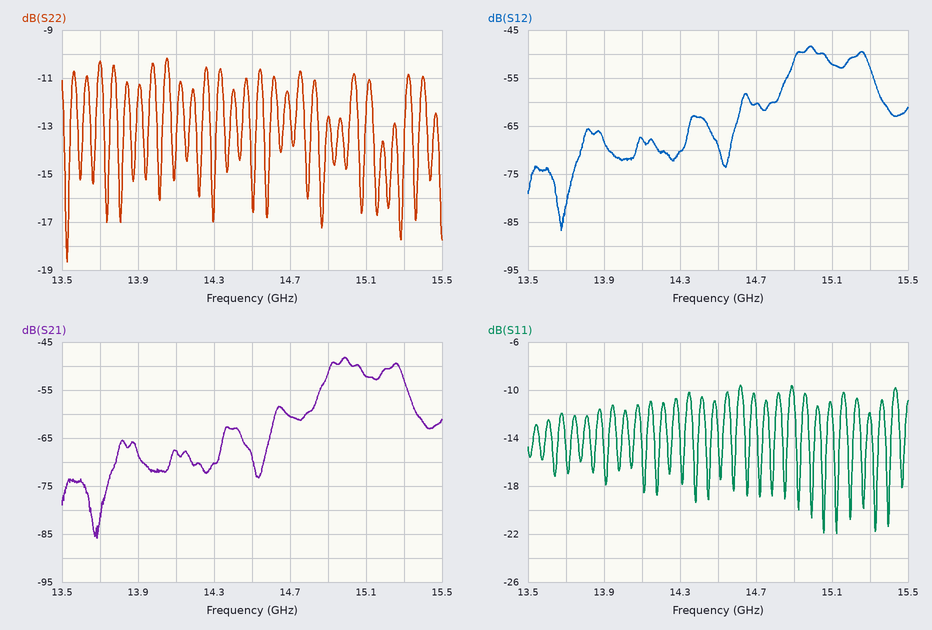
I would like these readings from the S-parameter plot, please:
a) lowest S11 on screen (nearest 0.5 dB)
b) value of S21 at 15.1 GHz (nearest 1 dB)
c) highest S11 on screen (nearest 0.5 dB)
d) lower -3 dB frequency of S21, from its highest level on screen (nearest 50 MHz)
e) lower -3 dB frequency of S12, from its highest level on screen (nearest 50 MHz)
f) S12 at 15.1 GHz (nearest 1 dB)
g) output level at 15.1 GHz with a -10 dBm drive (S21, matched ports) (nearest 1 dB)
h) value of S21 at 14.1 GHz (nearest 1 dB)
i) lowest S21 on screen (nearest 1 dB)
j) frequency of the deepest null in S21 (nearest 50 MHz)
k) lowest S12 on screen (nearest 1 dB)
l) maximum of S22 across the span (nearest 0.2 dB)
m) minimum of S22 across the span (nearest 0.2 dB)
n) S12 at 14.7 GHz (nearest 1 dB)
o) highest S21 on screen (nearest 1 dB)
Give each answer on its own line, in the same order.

-22.0 dB
-52 dB
-9.5 dB
14.90 GHz
14.90 GHz
-52 dB
-62 dBm
-68 dB
-86 dB
13.70 GHz
-87 dB
-10.2 dB
-18.6 dB
-60 dB
-48 dB
